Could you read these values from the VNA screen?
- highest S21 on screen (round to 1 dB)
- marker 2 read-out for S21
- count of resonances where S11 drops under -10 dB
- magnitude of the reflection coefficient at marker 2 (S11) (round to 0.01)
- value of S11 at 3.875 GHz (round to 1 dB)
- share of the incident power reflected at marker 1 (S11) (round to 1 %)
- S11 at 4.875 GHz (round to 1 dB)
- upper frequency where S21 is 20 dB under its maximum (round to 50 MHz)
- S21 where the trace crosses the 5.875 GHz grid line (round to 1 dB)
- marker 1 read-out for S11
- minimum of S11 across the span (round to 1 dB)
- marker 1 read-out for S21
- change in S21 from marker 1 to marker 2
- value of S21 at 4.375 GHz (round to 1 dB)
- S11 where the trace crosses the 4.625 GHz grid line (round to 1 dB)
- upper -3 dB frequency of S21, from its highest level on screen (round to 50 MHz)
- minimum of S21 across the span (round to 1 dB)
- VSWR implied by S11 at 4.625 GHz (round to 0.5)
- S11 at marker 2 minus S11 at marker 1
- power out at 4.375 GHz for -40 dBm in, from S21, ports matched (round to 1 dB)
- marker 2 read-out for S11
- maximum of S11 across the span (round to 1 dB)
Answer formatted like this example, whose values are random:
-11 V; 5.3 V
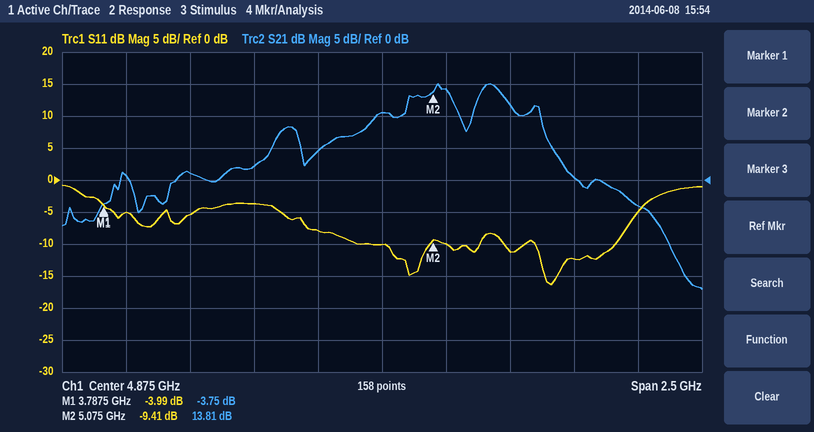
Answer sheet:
15 dB; 13.81 dB; 2; 0.34; -5 dB; 40 %; -10 dB; 5.90 GHz; -4 dB; -3.99 dB; -16 dB; -3.75 dB; 17.56 dB; 2 dB; -8 dB; 5.35 GHz; -17 dB; 2.5; -5.42 dB; -38 dBm; -9.41 dB; -1 dB
